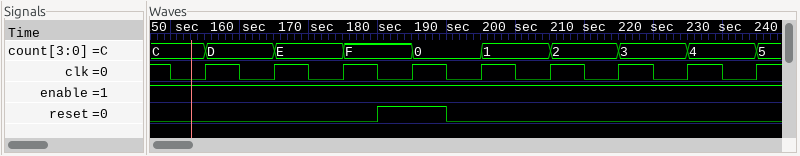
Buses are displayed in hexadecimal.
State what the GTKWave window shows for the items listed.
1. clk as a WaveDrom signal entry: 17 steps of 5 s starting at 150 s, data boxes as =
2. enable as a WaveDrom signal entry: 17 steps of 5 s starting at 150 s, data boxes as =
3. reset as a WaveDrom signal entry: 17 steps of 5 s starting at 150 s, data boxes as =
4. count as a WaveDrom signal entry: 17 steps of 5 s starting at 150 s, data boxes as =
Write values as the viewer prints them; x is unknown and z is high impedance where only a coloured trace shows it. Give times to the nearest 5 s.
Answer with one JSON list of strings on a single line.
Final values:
["{name: 'clk', wave: '01010101010101010'}", "{name: 'enable', wave: '1................'}", "{name: 'reset', wave: '0.....1.0........'}", "{name: 'count', wave: '==.=.=.=.=.=.=.=.', data: 'C D E F 0 1 2 3 4'}"]
